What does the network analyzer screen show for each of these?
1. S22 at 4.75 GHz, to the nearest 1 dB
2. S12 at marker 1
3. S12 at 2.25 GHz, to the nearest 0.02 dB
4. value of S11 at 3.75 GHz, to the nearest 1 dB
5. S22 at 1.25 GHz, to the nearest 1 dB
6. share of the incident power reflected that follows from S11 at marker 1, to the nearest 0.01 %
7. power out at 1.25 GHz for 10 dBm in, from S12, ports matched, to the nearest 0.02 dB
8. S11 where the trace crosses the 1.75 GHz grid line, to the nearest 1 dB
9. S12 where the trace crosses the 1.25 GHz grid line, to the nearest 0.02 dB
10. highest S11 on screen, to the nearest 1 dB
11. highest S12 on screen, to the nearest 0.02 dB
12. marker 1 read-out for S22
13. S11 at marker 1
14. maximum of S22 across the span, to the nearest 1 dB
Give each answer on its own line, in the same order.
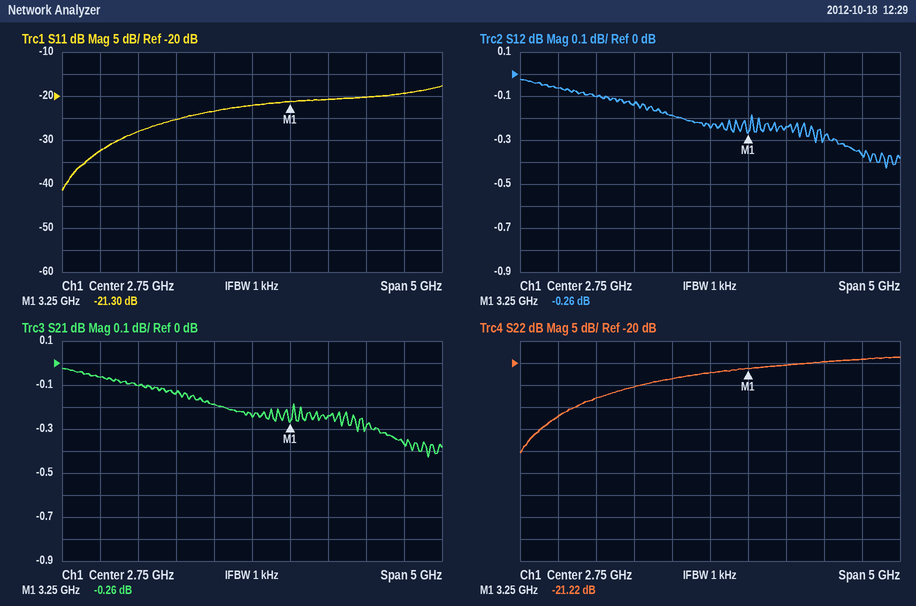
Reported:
-19 dB
-0.26 dB
-0.18 dB
-21 dB
-28 dB
0.74 %
9.90 dBm
-25 dB
-0.10 dB
-18 dB
-0.02 dB
-21.22 dB
-21.30 dB
-19 dB
